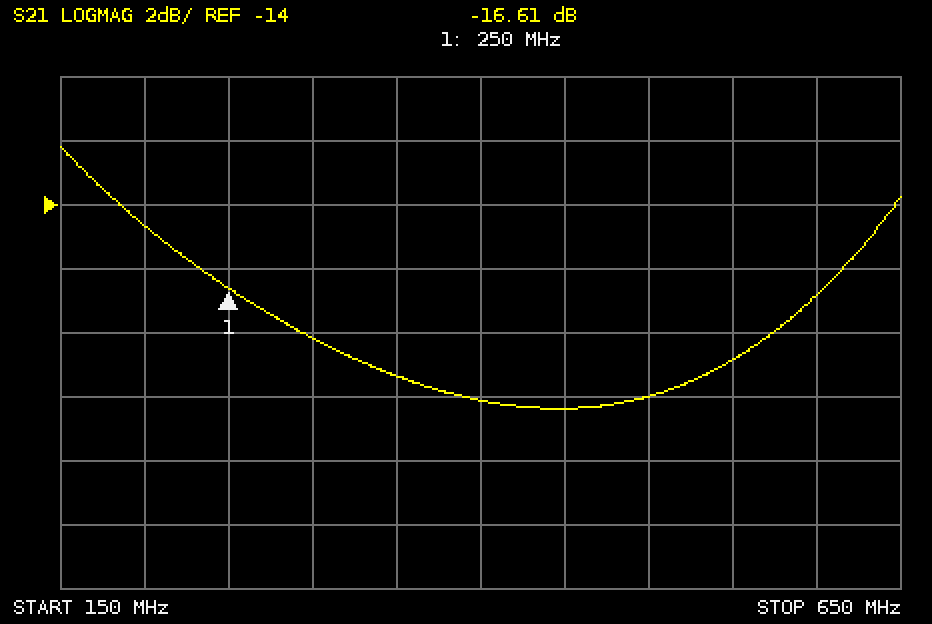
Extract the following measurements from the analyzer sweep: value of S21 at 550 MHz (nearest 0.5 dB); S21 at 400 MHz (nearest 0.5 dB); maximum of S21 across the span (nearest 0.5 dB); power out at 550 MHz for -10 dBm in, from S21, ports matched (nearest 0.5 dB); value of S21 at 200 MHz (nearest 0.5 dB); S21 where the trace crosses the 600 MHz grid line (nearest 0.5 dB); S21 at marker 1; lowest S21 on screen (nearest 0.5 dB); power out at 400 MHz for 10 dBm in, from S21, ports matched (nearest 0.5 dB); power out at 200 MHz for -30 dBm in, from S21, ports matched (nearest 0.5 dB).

-19.0 dB
-20.0 dB
-12.0 dB
-29.0 dBm
-14.5 dB
-17.0 dB
-16.61 dB
-20.5 dB
-10.0 dBm
-44.5 dBm
